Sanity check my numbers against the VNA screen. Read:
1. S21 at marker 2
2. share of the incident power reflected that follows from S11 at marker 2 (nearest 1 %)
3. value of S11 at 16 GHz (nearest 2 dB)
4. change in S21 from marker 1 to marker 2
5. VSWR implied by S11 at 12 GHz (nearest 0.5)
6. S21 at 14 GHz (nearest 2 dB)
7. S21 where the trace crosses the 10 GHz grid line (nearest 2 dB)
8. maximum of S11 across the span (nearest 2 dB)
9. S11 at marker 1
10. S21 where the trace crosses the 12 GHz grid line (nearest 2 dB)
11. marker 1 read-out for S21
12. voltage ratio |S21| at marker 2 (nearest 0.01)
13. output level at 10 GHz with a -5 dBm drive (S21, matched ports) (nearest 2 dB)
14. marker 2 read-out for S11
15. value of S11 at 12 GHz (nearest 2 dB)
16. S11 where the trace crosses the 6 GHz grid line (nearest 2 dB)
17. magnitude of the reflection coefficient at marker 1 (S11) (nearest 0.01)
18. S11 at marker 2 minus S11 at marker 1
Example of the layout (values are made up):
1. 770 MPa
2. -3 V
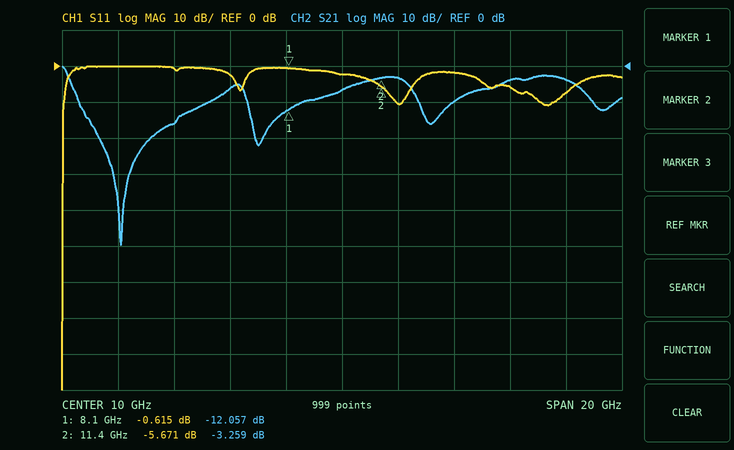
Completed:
1. -3.259 dB
2. 27 %
3. -6 dB
4. 8.798 dB
5. 2.0
6. -10 dB
7. -6 dB
8. 0 dB
9. -0.615 dB
10. -4 dB
11. -12.057 dB
12. 0.69
13. -12 dBm
14. -5.671 dB
15. -10 dB
16. -2 dB
17. 0.93
18. -5.056 dB
